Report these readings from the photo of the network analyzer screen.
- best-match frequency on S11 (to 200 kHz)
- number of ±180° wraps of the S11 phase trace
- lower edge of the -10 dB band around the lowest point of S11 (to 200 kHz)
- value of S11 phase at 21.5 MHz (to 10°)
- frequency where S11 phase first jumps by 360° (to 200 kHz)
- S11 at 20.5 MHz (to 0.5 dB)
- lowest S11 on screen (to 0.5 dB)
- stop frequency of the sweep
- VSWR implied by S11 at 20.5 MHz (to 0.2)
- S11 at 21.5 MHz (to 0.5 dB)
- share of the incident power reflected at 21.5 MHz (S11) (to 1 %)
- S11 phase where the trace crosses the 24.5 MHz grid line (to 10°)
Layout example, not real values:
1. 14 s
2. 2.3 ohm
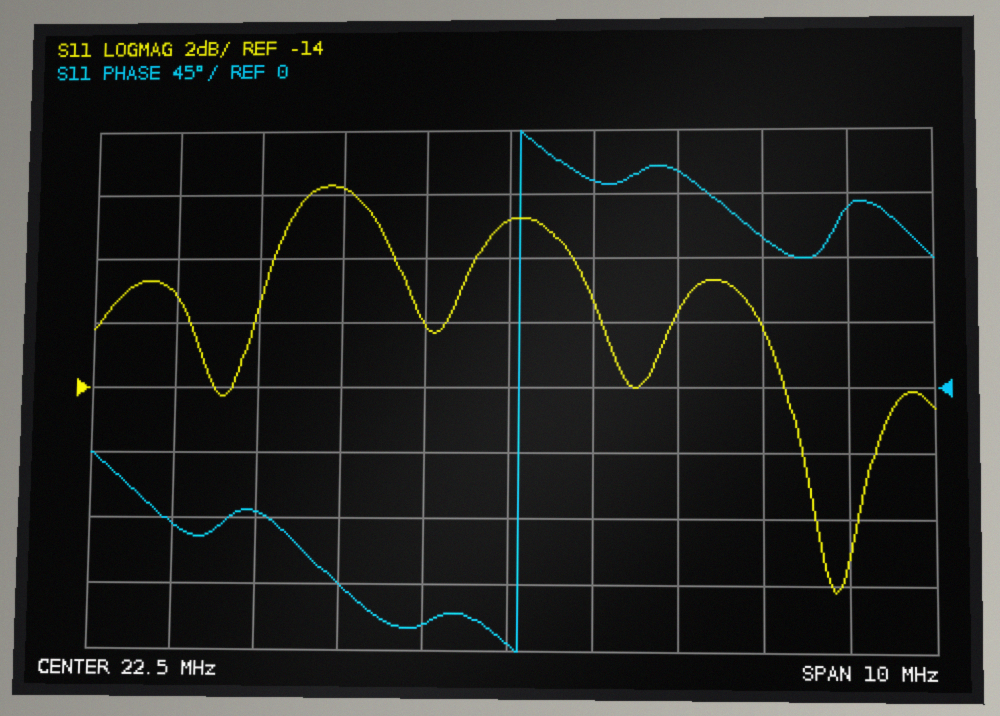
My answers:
1. 26.4 MHz
2. 1
3. 23.2 MHz
4. -160°
5. 22.6 MHz
6. -8.0 dB
7. -20.0 dB
8. 27.5 MHz
9. 2.4
10. -12.0 dB
11. 6 %
12. 150°
